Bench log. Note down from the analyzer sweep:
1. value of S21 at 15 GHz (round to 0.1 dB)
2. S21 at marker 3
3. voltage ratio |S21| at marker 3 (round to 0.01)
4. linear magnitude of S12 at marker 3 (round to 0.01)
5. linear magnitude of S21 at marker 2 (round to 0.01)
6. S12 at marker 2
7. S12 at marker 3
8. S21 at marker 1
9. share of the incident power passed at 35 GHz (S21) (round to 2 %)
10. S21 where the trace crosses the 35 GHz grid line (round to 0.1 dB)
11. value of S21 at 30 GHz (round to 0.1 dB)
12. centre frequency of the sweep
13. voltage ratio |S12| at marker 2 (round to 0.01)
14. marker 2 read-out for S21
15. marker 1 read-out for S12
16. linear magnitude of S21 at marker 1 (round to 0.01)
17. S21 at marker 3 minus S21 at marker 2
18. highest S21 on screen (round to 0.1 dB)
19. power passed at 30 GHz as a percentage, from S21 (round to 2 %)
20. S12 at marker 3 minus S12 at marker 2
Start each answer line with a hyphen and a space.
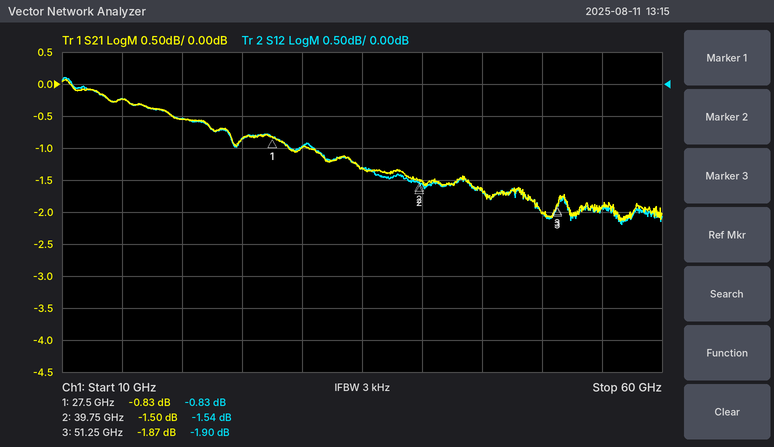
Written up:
- -0.2 dB
- -1.87 dB
- 0.81
- 0.80
- 0.84
- -1.54 dB
- -1.90 dB
- -0.83 dB
- 74 %
- -1.3 dB
- -1.0 dB
- 35 GHz
- 0.84
- -1.50 dB
- -0.83 dB
- 0.91
- -0.37 dB
- 0.1 dB
- 80 %
- -0.36 dB
